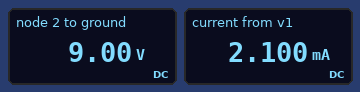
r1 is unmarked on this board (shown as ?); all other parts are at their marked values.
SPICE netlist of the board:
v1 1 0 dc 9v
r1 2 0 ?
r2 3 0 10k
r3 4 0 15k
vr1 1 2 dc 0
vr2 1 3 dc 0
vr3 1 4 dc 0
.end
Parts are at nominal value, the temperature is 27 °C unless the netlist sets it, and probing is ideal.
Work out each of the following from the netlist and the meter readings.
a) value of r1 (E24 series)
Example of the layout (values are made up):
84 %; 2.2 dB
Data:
15 kΩ
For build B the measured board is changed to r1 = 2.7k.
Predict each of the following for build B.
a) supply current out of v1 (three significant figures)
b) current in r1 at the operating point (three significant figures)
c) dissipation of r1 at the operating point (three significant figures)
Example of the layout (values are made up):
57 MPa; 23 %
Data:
4.83 mA; 3.33 mA; 30.0 mW
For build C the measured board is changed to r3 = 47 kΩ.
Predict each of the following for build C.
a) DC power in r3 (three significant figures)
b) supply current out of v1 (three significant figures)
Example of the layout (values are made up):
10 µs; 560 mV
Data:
1.72 mW; 1.69 mA
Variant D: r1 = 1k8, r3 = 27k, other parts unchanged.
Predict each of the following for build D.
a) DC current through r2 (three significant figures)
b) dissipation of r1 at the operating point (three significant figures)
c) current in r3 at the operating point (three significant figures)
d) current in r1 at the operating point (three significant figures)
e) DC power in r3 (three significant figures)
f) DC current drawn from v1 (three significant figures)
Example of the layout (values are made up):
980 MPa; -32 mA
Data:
900 µA; 45.0 mW; 333 µA; 5.00 mA; 3.00 mW; 6.23 mA
